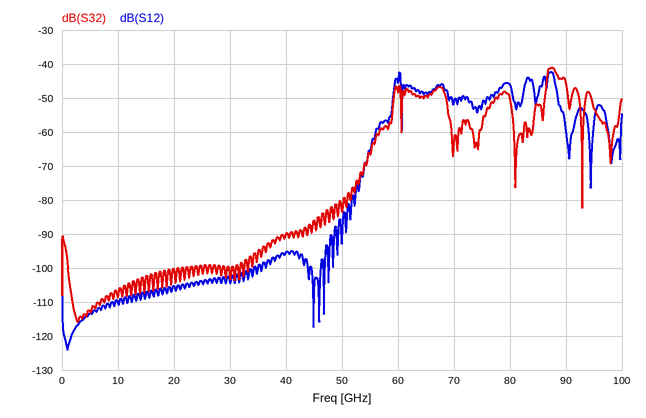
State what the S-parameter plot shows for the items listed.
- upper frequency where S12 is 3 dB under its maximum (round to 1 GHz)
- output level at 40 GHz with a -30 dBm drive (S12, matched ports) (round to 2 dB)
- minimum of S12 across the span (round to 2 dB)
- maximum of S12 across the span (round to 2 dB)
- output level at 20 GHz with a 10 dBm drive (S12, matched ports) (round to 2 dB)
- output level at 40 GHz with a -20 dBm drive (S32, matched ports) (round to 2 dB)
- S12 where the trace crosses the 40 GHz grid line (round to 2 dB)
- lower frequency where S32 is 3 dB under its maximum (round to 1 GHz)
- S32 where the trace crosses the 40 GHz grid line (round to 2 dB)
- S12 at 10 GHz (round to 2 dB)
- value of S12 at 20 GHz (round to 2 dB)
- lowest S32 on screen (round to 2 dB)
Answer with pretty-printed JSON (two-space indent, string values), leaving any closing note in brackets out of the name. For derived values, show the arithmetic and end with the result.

{
  "upper frequency where S12 is 3 dB under its maximum": "88 GHz",
  "output level at 40 GHz with a -30 dBm drive (S12, matched ports)": "-30 dBm + (-96 dB) = -126 dBm",
  "minimum of S12 across the span": "-124 dB",
  "maximum of S12 across the span": "-42 dB",
  "output level at 20 GHz with a 10 dBm drive (S12, matched ports)": "10 dBm + (-106 dB) = -96 dBm",
  "output level at 40 GHz with a -20 dBm drive (S32, matched ports)": "-20 dBm + (-90 dB) = -110 dBm",
  "S12 where the trace crosses the 40 GHz grid line": "-96 dB",
  "lower frequency where S32 is 3 dB under its maximum": "87 GHz",
  "S32 where the trace crosses the 40 GHz grid line": "-90 dB",
  "S12 at 10 GHz": "-110 dB",
  "value of S12 at 20 GHz": "-106 dB",
  "lowest S32 on screen": "-116 dB"
}
